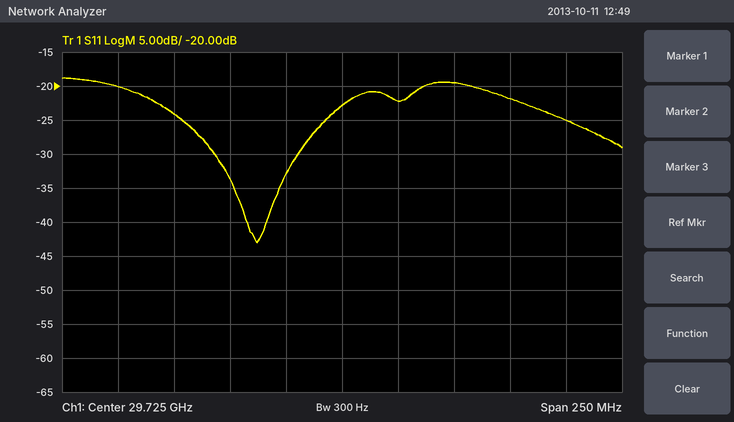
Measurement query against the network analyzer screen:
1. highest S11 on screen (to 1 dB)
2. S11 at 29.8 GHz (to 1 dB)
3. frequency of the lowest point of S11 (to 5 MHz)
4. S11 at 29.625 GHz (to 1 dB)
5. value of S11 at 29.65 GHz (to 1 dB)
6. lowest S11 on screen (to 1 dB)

-19 dB
-22 dB
29.685 GHz
-20 dB
-24 dB
-43 dB
